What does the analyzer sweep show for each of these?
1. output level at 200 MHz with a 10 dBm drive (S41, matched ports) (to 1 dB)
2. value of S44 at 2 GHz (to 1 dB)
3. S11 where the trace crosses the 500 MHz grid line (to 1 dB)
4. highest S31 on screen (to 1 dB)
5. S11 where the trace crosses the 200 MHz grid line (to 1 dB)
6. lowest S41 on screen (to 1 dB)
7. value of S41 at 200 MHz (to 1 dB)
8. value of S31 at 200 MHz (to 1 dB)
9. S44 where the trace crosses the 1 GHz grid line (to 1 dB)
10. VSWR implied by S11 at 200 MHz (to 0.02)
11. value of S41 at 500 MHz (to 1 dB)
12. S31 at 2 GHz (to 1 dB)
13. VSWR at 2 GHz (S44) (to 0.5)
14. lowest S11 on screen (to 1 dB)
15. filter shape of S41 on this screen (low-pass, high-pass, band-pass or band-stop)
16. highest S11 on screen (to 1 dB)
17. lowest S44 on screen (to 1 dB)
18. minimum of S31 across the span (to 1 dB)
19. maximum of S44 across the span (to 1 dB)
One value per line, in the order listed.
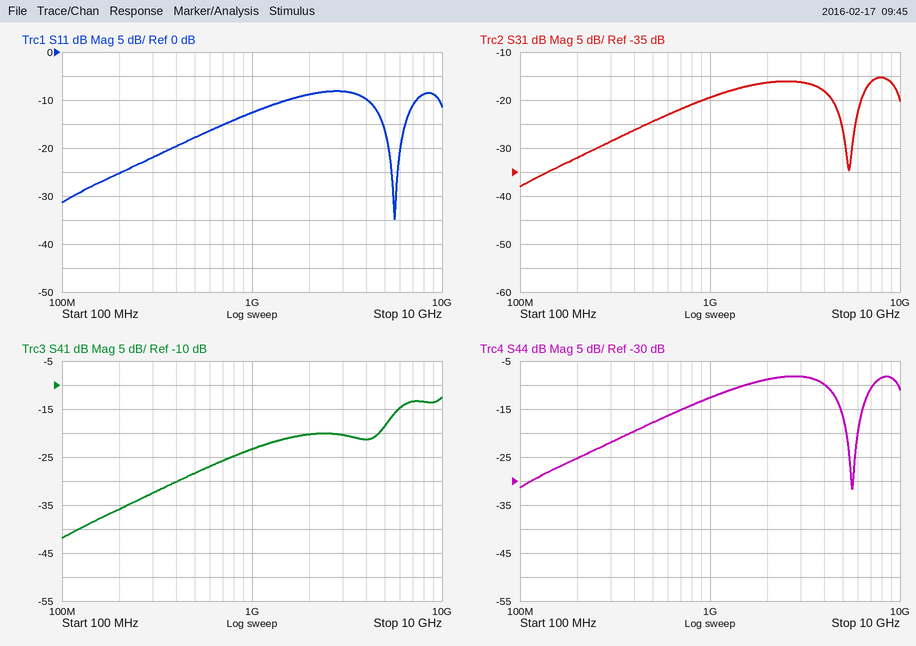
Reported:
-26 dBm
-9 dB
-18 dB
-15 dB
-25 dB
-42 dB
-36 dB
-32 dB
-13 dB
1.12
-28 dB
-16 dB
2.0
-35 dB
high-pass
-8 dB
-32 dB
-38 dB
-8 dB
